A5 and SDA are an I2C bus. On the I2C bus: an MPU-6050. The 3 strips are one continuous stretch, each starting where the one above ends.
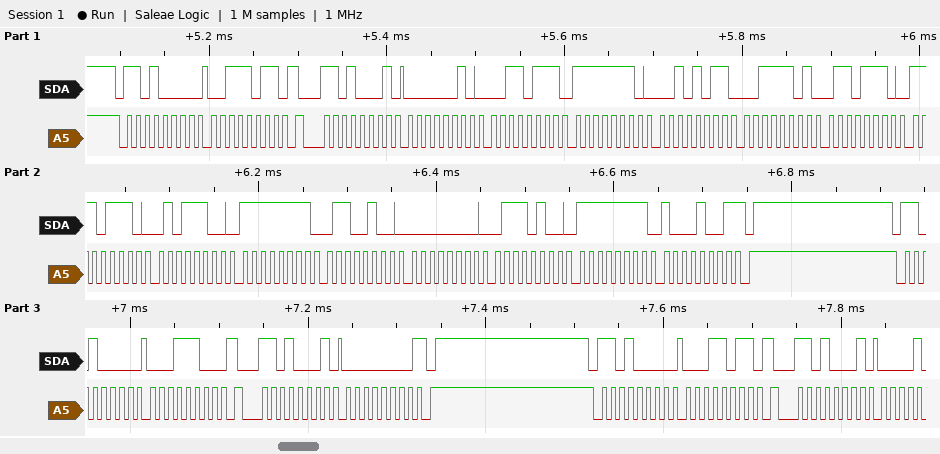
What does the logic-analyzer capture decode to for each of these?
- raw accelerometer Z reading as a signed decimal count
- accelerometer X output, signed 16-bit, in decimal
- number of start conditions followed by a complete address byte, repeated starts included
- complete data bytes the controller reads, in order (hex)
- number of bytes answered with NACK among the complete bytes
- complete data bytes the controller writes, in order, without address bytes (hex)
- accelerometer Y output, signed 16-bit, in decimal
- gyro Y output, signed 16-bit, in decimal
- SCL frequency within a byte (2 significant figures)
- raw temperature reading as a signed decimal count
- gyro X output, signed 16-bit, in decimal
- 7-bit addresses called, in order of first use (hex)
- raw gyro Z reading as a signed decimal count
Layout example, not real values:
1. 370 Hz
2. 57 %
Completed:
1. 15726
2. 567
3. 6
4. 02 37 FE 2B 3D 6E EE 5C FF 64 00 74 FF 89 00
5. 2
6. 3B 1C 1B
7. -469
8. 116
9. 100 kHz
10. -4516
11. -156
12. 0x68
13. -119
